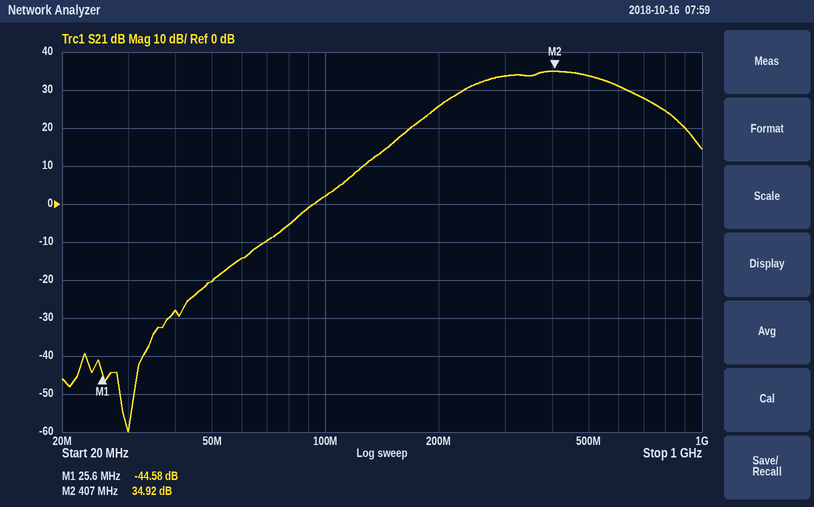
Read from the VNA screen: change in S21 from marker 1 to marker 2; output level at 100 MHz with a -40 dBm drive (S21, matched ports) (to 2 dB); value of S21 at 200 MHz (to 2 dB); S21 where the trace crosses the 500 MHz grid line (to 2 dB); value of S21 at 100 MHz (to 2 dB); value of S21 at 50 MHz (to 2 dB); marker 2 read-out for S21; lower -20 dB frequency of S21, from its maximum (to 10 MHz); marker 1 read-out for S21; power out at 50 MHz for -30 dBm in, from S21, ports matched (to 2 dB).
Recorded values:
79.50 dB
-38 dBm
26 dB
34 dB
2 dB
-20 dB
34.92 dB
150 MHz
-44.58 dB
-50 dBm
